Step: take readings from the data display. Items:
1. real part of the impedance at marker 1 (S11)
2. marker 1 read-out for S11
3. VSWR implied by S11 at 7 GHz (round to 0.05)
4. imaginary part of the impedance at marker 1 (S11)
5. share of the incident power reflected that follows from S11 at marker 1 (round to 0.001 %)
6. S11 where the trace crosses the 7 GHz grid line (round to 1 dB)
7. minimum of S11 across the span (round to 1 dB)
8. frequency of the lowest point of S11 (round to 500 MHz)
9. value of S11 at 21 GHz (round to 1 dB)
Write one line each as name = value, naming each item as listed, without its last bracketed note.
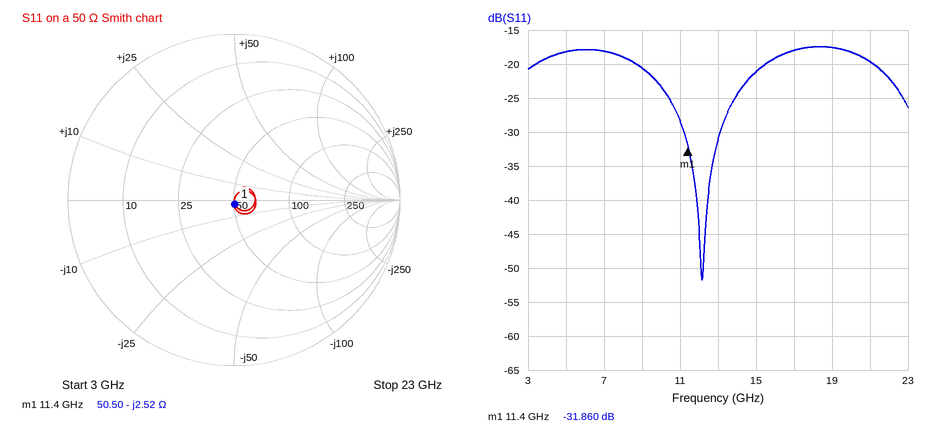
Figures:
real part of the impedance at marker 1 = 50.50 Ω
marker 1 read-out for S11 = -31.860 dB
VSWR implied by S11 at 7 GHz = 1.30
imaginary part of the impedance at marker 1 = -2.52 Ω
share of the incident power reflected that follows from S11 at marker 1 = 0.065 %
S11 where the trace crosses the 7 GHz grid line = -18 dB
minimum of S11 across the span = -52 dB
frequency of the lowest point of S11 = 12.0 GHz
value of S11 at 21 GHz = -20 dB
